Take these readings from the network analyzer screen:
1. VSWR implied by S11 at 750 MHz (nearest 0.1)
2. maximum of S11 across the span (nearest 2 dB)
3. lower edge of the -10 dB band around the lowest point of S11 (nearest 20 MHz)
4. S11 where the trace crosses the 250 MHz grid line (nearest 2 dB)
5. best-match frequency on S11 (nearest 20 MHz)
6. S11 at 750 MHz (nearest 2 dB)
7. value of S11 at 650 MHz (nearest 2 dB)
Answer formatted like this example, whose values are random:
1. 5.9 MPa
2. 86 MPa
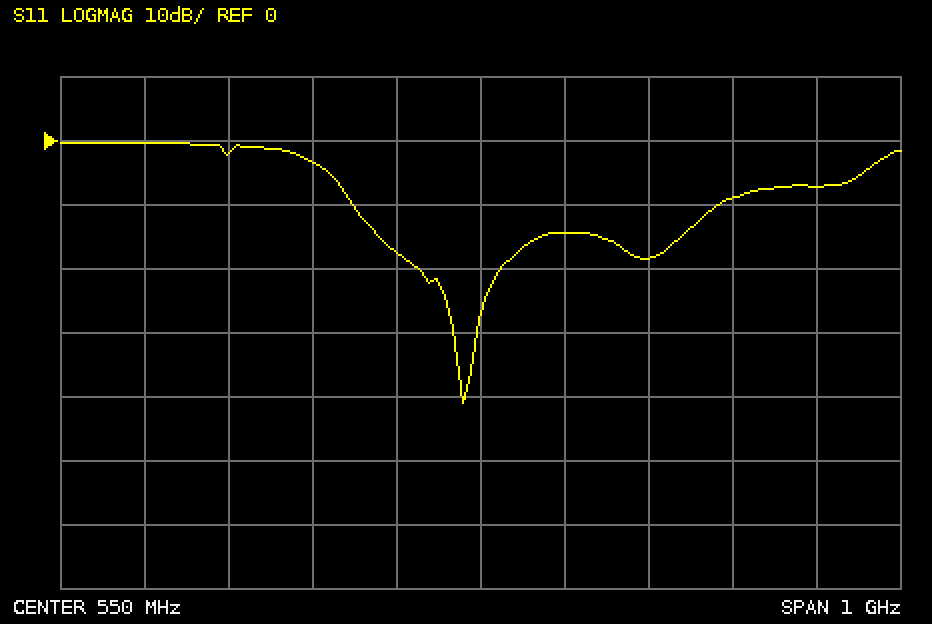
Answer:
1. 1.3
2. 0 dB
3. 400 MHz
4. -2 dB
5. 520 MHz
6. -18 dB
7. -14 dB
